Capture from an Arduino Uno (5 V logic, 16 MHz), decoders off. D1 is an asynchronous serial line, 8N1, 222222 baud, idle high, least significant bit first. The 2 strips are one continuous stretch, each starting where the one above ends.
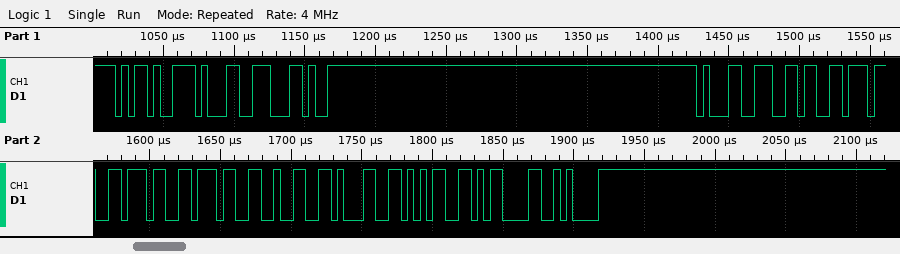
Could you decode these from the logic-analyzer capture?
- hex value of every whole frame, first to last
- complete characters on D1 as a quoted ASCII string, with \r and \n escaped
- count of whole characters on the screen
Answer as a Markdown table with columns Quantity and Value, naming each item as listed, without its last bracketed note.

| Quantity | Value |
|---|---|
| hex value of every whole frame, first to last | 2D 31 2C 31 36 37 37 37 32 31 35 0D 0A |
| complete characters on D1 as a quoted ASCII string, with \r and \n escaped | "-1,16777215\r\n" |
| count of whole characters on the screen | 13 |
